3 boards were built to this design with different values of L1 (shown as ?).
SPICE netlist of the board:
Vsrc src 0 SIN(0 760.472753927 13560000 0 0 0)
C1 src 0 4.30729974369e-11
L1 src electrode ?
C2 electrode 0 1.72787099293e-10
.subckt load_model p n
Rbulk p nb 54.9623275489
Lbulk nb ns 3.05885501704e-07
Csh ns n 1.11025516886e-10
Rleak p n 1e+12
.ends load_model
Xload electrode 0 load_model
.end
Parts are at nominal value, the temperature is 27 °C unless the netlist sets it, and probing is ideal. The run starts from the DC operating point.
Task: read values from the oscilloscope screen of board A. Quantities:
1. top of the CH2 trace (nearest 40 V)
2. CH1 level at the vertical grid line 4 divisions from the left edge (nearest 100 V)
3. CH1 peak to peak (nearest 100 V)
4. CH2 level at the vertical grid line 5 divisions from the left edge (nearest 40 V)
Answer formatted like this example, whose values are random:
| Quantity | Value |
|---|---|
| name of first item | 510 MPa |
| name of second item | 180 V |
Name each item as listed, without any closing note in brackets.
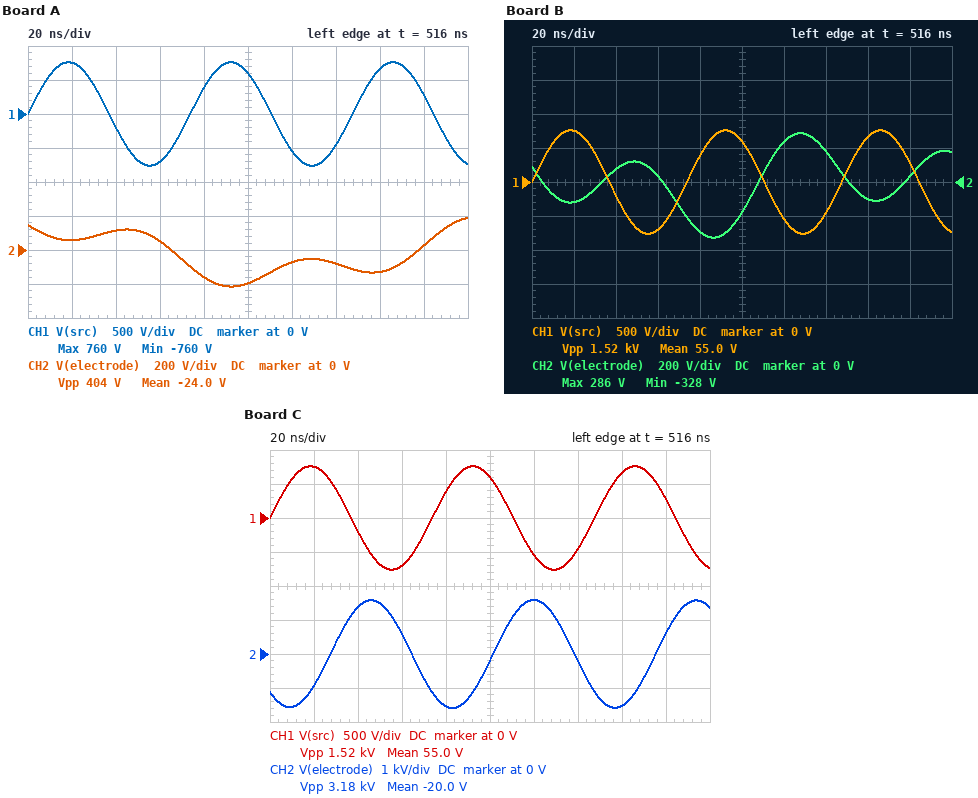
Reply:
| Quantity | Value |
|---|---|
| top of the CH2 trace | 200 V |
| CH1 level at the vertical grid line 4 divisions from the left edge | 400 V |
| CH1 peak to peak | 1.5 kV |
| CH2 level at the vertical grid line 5 divisions from the left edge | -200 V |
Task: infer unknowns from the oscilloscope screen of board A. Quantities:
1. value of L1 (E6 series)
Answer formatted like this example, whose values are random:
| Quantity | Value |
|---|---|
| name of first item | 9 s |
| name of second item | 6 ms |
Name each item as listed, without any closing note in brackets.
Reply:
| Quantity | Value |
|---|---|
| value of L1 | 4.7 µH |
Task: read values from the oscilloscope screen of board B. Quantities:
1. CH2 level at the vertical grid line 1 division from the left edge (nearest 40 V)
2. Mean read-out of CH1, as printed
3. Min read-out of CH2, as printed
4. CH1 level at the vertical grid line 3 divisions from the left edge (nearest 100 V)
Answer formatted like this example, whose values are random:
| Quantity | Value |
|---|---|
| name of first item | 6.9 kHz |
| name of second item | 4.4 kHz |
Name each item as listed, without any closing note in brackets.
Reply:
| Quantity | Value |
|---|---|
| CH2 level at the vertical grid line 1 division from the left edge | -120 V |
| Mean read-out of CH1, as printed | 55.0 V |
| Min read-out of CH2, as printed | -328 V |
| CH1 level at the vertical grid line 3 divisions from the left edge | -700 V |
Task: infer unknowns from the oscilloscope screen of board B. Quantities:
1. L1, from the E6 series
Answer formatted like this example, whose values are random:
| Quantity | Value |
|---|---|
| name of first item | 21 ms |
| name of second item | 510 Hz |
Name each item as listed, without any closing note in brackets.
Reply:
| Quantity | Value |
|---|---|
| L1, from the E6 series | 2.2 µH |
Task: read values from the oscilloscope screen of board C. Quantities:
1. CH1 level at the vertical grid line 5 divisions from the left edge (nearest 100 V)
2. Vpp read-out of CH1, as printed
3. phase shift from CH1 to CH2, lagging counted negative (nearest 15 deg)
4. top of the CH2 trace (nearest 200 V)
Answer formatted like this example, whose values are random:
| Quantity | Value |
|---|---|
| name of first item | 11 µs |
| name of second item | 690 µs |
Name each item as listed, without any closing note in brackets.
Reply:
| Quantity | Value |
|---|---|
| CH1 level at the vertical grid line 5 divisions from the left edge | 600 V |
| Vpp read-out of CH1, as printed | 1.52 kV |
| phase shift from CH1 to CH2, lagging counted negative | -135 deg |
| top of the CH2 trace | 1.6 kV |
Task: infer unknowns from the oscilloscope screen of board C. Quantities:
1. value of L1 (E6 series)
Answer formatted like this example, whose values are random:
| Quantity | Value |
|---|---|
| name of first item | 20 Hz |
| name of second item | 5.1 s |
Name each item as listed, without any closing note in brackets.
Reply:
| Quantity | Value |
|---|---|
| value of L1 | 680 nH |
